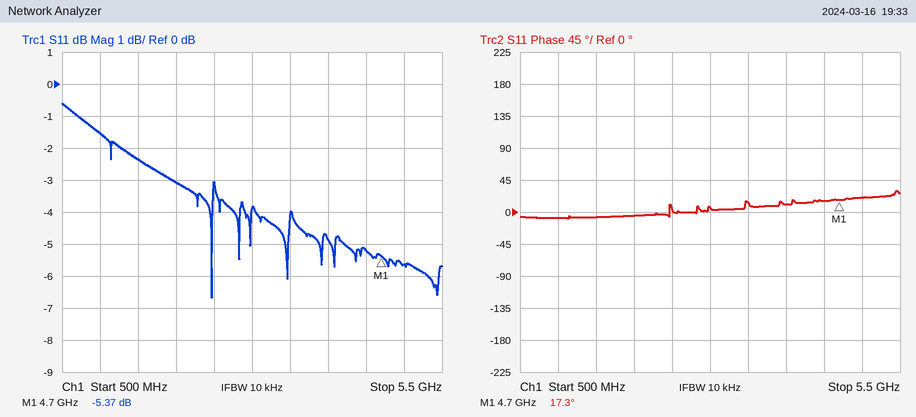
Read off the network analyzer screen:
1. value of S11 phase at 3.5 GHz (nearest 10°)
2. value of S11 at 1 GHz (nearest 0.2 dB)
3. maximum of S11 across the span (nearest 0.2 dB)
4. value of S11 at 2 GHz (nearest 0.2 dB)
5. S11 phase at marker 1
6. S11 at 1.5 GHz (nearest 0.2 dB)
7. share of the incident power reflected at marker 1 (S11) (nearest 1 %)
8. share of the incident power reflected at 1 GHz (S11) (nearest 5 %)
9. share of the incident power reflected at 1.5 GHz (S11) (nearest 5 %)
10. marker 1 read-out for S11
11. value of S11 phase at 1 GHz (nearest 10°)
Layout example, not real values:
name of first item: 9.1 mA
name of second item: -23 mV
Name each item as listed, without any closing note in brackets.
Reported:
value of S11 phase at 3.5 GHz: 10°
value of S11 at 1 GHz: -1.6 dB
maximum of S11 across the span: -0.6 dB
value of S11 at 2 GHz: -3.0 dB
S11 phase at marker 1: 17.3°
S11 at 1.5 GHz: -2.4 dB
share of the incident power reflected at marker 1 (S11): 29 %
share of the incident power reflected at 1 GHz (S11): 70 %
share of the incident power reflected at 1.5 GHz (S11): 60 %
marker 1 read-out for S11: -5.37 dB
value of S11 phase at 1 GHz: -10°
